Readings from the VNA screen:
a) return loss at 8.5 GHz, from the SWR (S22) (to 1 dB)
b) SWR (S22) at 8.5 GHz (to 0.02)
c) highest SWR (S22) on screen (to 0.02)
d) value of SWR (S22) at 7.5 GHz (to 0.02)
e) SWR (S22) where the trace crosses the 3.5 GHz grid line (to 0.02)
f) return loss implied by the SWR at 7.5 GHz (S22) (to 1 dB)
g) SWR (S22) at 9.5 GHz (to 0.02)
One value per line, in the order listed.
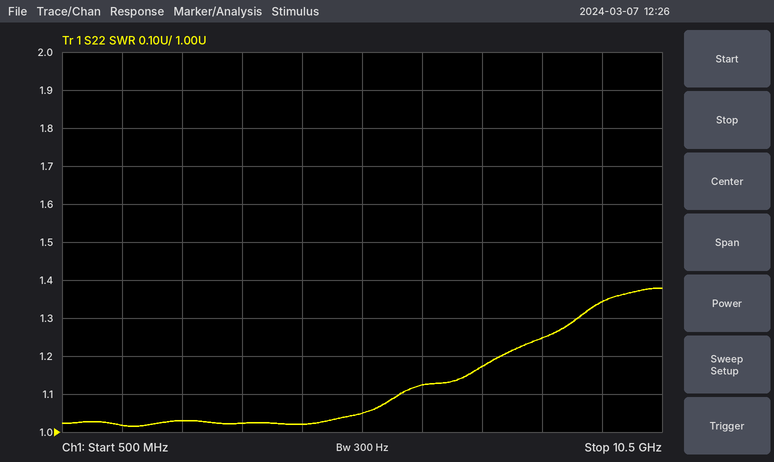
19 dB
1.24
1.38
1.18
1.02
22 dB
1.34
